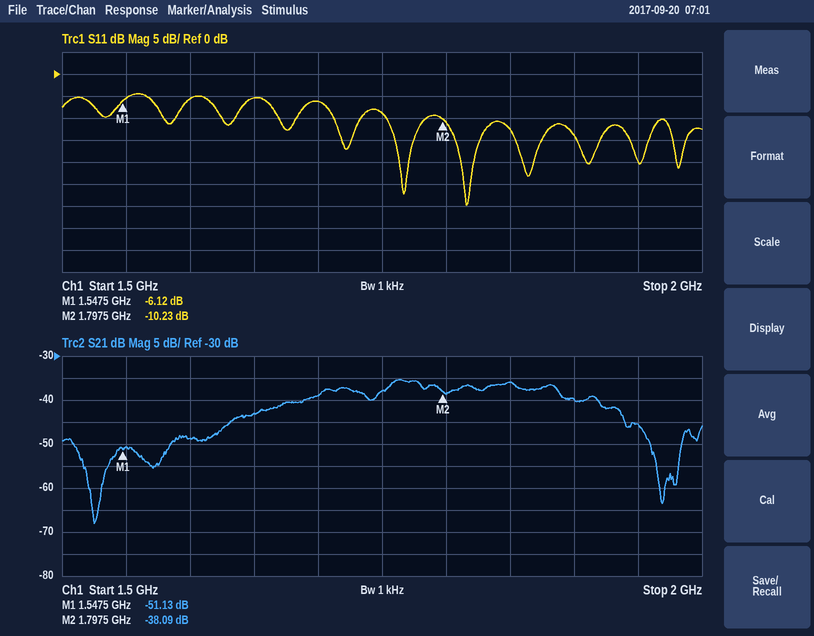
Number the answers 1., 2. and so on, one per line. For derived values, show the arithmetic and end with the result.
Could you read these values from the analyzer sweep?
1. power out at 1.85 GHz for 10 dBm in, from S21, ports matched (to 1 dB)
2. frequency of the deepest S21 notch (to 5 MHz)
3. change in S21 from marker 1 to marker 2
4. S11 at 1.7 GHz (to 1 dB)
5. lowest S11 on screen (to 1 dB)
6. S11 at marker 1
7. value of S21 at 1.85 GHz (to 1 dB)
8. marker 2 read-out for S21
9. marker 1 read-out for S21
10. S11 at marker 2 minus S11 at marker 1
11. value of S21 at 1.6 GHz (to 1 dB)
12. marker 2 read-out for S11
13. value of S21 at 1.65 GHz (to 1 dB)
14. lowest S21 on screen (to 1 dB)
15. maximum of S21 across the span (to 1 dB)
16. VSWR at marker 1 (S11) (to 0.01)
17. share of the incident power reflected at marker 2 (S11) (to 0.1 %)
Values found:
1. 10 dBm + (-36 dB) = -26 dBm
2. 1.525 GHz
3. -38.09 − (-51.13) = 13.04 dB
4. -6 dB
5. -30 dB
6. -6.12 dB
7. -36 dB
8. -38.09 dB
9. -51.13 dB
10. -10.23 − (-6.12) = -4.11 dB
11. -49 dB
12. -10.23 dB
13. -43 dB
14. -68 dB
15. -35 dB
16. (1 + 0.4943)/(1 − 0.4943) ≈ 2.95
17. 10^(-10.23/10) ≈ 9.5 %
